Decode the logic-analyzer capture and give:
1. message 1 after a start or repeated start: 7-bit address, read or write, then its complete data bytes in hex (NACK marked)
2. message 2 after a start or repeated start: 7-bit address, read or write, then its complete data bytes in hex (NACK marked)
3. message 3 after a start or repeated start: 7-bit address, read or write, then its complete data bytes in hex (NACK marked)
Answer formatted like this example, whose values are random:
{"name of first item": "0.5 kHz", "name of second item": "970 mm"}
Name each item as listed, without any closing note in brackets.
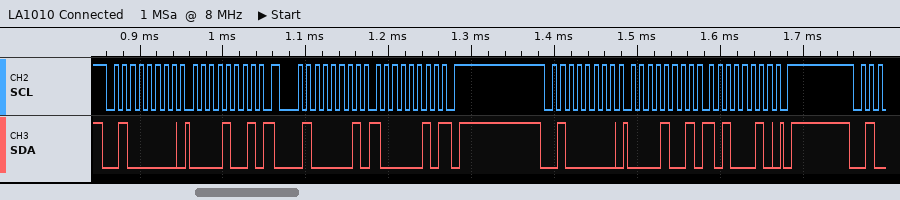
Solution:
{"message 1 after a start or repeated start: 7-bit address, read or write, then its complete data bytes in hex": "0x20 write: 09", "message 2 after a start or repeated start: 7-bit address, read or write, then its complete data bytes in hex": "0x20 read: 82 NACK", "message 3 after a start or repeated start: 7-bit address, read or write, then its complete data bytes in hex": "0x20 write: 09 A2"}
